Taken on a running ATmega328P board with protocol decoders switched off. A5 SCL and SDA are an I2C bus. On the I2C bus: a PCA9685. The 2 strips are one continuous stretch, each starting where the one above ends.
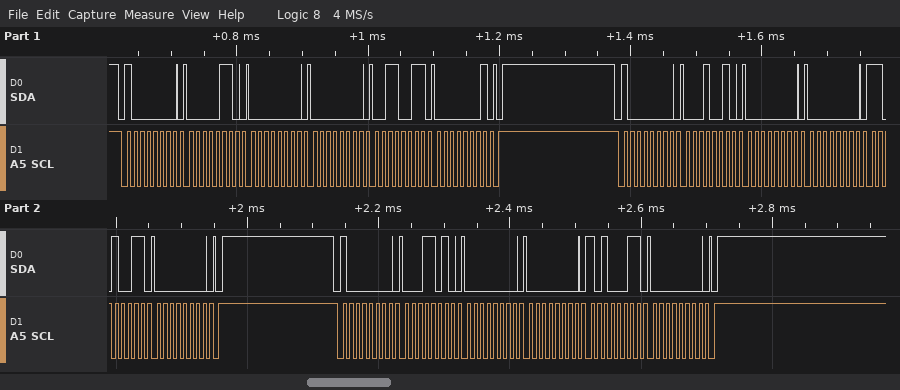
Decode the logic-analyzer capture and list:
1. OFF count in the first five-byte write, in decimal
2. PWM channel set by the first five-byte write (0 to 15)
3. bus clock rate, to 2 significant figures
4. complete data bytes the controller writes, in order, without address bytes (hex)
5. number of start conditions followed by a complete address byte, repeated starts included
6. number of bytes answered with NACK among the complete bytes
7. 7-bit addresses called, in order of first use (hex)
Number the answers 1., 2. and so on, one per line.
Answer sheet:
1. 307
2. 0
3. 100 kHz
4. 06 00 00 33 01 12 00 00 D3 00 1A 00 00 A3 00
5. 3
6. 0
7. 0x40
